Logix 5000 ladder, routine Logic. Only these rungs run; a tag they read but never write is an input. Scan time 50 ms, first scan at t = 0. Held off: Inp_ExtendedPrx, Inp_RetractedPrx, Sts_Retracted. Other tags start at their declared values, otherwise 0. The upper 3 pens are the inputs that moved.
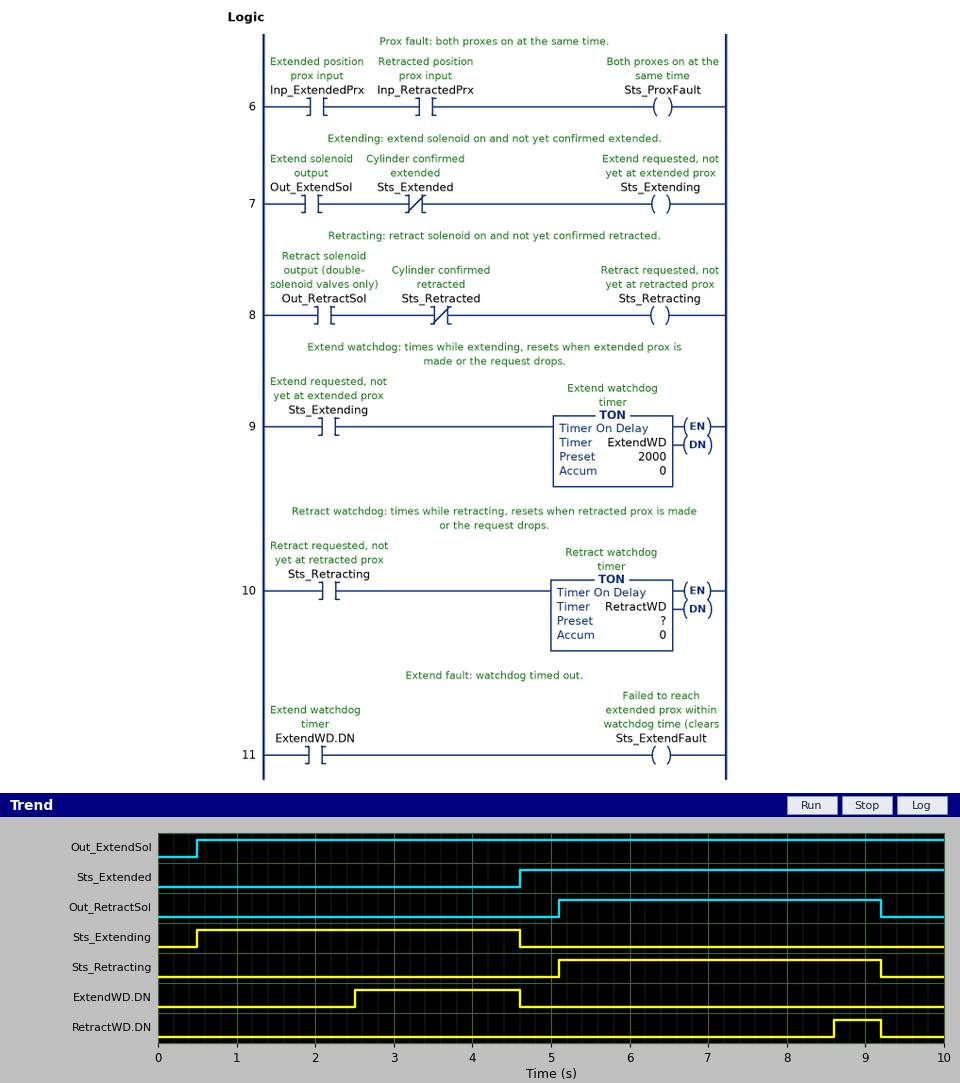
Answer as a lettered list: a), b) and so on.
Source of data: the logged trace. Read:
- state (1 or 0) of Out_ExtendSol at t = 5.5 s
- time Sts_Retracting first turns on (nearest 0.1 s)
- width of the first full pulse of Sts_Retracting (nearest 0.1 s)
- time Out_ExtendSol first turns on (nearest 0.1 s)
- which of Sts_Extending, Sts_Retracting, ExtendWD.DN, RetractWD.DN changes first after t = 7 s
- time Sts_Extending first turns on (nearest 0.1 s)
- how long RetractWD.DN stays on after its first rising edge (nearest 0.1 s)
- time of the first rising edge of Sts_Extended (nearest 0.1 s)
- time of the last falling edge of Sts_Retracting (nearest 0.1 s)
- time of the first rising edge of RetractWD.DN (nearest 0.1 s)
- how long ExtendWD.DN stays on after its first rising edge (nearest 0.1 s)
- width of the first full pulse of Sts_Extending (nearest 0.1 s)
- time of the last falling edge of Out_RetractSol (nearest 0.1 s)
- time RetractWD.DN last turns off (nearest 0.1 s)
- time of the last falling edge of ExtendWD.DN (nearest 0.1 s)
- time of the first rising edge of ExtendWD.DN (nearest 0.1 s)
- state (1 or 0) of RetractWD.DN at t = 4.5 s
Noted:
a) 1
b) 5.1 s
c) 4.1 s
d) 0.5 s
e) RetractWD.DN
f) 0.5 s
g) 0.6 s
h) 4.6 s
i) 9.2 s
j) 8.6 s
k) 2.1 s
l) 4.1 s
m) 9.2 s
n) 9.2 s
o) 4.6 s
p) 2.5 s
q) 0
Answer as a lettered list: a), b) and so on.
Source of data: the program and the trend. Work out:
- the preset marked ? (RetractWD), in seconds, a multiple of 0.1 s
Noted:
a) 3.5 s
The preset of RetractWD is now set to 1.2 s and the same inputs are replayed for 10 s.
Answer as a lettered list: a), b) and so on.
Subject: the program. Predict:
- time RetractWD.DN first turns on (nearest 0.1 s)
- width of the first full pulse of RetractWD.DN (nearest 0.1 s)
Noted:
a) 6.3 s
b) 2.9 s
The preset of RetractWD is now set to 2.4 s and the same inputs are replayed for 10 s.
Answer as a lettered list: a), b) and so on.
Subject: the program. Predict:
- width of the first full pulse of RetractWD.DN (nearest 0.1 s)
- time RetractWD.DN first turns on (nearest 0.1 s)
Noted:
a) 1.7 s
b) 7.5 s
